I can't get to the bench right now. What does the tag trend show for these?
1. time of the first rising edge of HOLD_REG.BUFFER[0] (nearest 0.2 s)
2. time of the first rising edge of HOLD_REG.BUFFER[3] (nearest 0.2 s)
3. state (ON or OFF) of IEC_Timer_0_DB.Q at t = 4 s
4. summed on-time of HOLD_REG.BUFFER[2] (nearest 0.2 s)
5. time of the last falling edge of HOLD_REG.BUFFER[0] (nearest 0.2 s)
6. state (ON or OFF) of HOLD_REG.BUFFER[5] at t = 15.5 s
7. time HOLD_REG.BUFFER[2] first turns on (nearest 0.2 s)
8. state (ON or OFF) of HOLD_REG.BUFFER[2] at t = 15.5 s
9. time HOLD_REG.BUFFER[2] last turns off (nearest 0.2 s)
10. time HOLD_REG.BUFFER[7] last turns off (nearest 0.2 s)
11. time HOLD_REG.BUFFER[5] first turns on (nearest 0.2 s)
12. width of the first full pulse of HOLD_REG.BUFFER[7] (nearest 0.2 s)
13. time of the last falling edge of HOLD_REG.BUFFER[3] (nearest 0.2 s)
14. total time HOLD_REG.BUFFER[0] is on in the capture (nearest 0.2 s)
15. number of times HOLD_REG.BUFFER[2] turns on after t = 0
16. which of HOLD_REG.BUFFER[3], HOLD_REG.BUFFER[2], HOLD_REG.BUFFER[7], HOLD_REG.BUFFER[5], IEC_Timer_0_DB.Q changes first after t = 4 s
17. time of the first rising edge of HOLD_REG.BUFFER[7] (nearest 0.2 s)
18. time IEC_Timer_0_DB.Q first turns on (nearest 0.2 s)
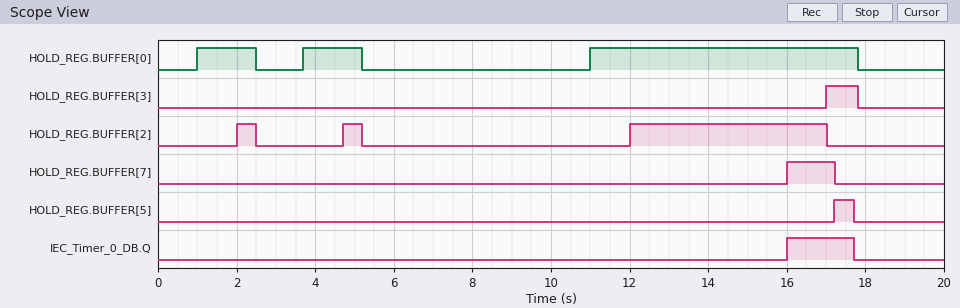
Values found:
1.0 s
17.0 s
OFF
6.0 s
17.8 s
OFF
2.0 s
ON
17.0 s
17.2 s
17.2 s
1.2 s
17.8 s
9.8 s
3
HOLD_REG.BUFFER[2]
16.0 s
16.0 s
